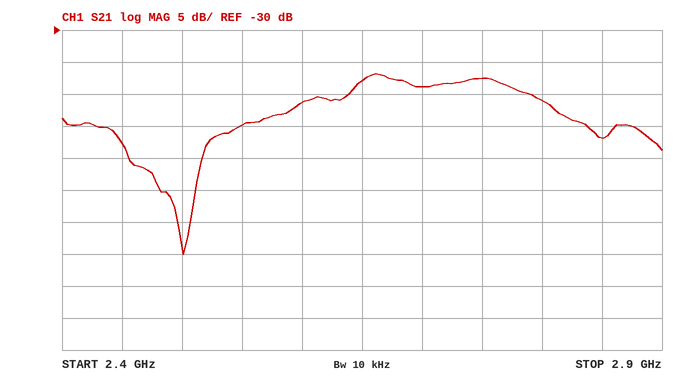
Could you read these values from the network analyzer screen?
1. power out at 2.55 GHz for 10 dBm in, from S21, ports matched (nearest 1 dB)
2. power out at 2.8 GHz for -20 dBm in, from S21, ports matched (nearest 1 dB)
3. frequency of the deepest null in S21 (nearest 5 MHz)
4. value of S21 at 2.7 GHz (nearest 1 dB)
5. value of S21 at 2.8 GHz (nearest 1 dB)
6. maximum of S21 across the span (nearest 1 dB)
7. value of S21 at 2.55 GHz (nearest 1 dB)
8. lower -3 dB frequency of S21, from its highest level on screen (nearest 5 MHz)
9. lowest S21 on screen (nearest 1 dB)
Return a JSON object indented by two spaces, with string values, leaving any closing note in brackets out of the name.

{
  "power out at 2.55 GHz for 10 dBm in, from S21, ports matched": "-35 dBm",
  "power out at 2.8 GHz for -20 dBm in, from S21, ports matched": "-61 dBm",
  "frequency of the deepest null in S21": "2.500 GHz",
  "value of S21 at 2.7 GHz": "-39 dB",
  "value of S21 at 2.8 GHz": "-41 dB",
  "maximum of S21 across the span": "-37 dB",
  "value of S21 at 2.55 GHz": "-45 dB",
  "lower -3 dB frequency of S21, from its highest level on screen": "2.640 GHz",
  "lowest S21 on screen": "-65 dB"
}
